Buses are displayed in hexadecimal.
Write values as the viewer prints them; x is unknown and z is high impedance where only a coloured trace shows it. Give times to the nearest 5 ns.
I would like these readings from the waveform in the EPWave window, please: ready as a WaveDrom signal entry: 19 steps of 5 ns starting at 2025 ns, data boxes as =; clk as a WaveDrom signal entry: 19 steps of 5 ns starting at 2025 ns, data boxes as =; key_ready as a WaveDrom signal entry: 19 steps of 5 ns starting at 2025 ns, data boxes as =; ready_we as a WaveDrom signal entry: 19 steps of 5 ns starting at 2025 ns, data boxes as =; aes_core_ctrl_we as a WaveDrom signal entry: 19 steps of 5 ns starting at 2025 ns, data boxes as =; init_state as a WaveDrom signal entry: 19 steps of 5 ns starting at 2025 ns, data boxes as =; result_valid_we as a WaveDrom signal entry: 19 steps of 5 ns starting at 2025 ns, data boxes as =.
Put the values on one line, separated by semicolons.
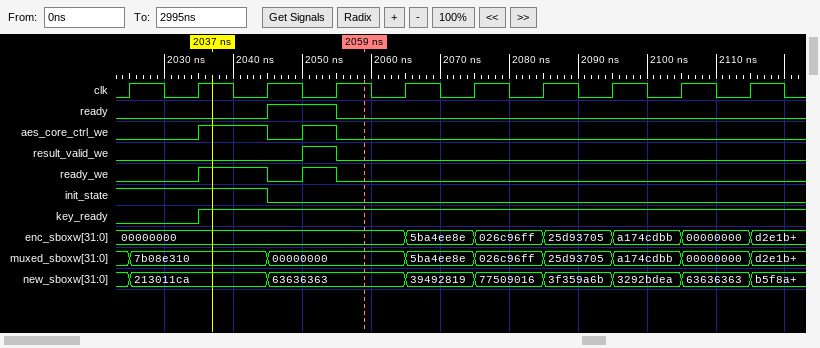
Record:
{name: 'ready', wave: '0...1.0............'}; {name: 'clk', wave: '1010101010101010101'}; {name: 'key_ready', wave: '0.1................'}; {name: 'ready_we', wave: '0.1.010............'}; {name: 'aes_core_ctrl_we', wave: '0.1.010............'}; {name: 'init_state', wave: '1...0..............'}; {name: 'result_valid_we', wave: '0....10............'}
